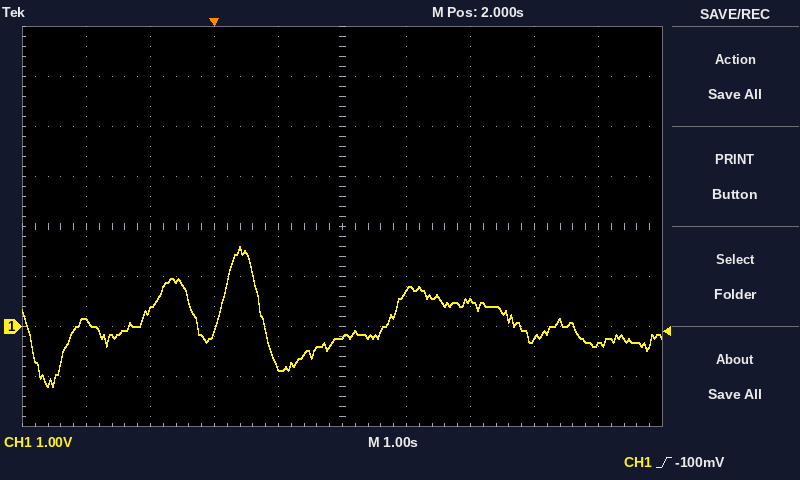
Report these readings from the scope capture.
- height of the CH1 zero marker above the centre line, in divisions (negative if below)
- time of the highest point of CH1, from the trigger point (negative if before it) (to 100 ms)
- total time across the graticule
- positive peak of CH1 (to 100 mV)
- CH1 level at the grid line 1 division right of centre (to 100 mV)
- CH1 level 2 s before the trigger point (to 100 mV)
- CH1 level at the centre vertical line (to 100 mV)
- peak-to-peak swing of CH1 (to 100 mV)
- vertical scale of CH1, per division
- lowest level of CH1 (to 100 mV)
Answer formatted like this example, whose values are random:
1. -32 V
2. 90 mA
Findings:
1. -2.0 div
2. +400 ms
3. 10 s
4. 1.6 V
5. 700 mV
6. 100 mV
7. -200 mV
8. 2.8 V
9. 1 V
10. -1.2 V
